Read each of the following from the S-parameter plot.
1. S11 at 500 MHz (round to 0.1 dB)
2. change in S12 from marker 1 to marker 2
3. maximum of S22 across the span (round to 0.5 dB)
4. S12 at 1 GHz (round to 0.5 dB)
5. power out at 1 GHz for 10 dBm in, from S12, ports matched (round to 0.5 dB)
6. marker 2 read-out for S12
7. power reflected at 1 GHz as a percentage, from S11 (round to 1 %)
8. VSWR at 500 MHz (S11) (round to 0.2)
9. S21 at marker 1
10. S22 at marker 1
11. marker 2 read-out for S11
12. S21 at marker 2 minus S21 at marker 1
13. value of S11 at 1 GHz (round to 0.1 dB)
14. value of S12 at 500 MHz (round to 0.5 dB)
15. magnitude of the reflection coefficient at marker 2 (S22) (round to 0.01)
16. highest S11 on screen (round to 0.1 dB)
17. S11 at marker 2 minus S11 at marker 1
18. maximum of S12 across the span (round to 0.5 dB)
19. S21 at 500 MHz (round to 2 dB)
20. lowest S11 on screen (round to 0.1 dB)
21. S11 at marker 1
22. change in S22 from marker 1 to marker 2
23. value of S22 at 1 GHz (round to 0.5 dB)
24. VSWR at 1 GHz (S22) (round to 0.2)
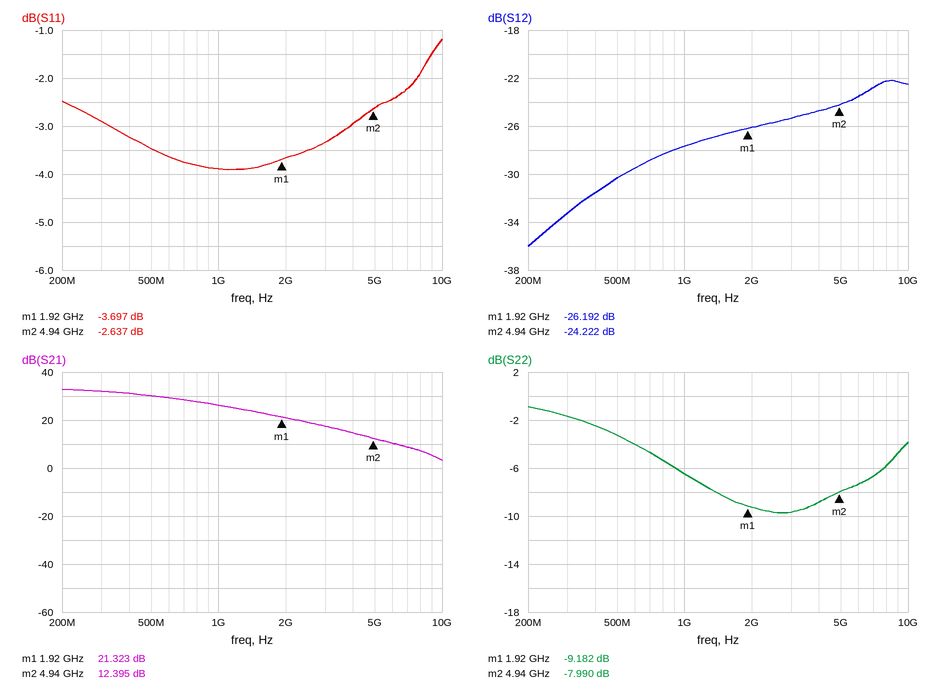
-3.5 dB
1.970 dB
-1.0 dB
-27.5 dB
-17.5 dBm
-24.222 dB
41 %
5.0
21.323 dB
-9.182 dB
-2.637 dB
-8.928 dB
-3.9 dB
-30.5 dB
0.40
-1.2 dB
1.060 dB
-22.0 dB
30 dB
-3.9 dB
-3.697 dB
1.192 dB
-6.5 dB
2.8
